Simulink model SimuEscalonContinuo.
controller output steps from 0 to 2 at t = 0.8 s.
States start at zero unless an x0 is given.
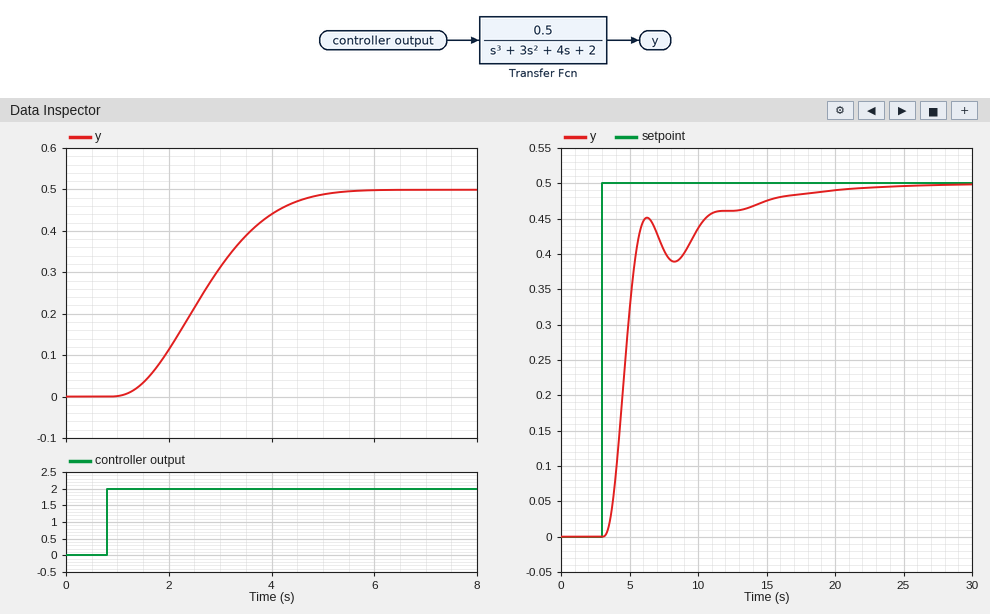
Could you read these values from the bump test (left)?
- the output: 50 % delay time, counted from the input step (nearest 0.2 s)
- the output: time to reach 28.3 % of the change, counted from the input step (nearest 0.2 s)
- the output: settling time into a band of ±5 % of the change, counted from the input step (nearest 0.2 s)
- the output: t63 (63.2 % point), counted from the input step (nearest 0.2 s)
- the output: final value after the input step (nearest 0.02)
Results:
1.8 s
1.4 s
3.8 s
2.2 s
0.50
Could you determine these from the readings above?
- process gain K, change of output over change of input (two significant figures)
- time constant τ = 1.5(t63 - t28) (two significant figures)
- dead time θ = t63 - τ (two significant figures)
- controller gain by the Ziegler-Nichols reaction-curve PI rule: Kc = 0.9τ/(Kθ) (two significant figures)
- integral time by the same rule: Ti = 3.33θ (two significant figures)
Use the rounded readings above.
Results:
0.25
1.2 s
1.0 s
4.3
3.3 s
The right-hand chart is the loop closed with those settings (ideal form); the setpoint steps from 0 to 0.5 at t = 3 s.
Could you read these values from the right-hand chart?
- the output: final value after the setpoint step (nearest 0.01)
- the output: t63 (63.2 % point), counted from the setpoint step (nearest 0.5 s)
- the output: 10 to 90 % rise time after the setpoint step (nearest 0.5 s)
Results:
0.50
2.0 s
2.5 s
